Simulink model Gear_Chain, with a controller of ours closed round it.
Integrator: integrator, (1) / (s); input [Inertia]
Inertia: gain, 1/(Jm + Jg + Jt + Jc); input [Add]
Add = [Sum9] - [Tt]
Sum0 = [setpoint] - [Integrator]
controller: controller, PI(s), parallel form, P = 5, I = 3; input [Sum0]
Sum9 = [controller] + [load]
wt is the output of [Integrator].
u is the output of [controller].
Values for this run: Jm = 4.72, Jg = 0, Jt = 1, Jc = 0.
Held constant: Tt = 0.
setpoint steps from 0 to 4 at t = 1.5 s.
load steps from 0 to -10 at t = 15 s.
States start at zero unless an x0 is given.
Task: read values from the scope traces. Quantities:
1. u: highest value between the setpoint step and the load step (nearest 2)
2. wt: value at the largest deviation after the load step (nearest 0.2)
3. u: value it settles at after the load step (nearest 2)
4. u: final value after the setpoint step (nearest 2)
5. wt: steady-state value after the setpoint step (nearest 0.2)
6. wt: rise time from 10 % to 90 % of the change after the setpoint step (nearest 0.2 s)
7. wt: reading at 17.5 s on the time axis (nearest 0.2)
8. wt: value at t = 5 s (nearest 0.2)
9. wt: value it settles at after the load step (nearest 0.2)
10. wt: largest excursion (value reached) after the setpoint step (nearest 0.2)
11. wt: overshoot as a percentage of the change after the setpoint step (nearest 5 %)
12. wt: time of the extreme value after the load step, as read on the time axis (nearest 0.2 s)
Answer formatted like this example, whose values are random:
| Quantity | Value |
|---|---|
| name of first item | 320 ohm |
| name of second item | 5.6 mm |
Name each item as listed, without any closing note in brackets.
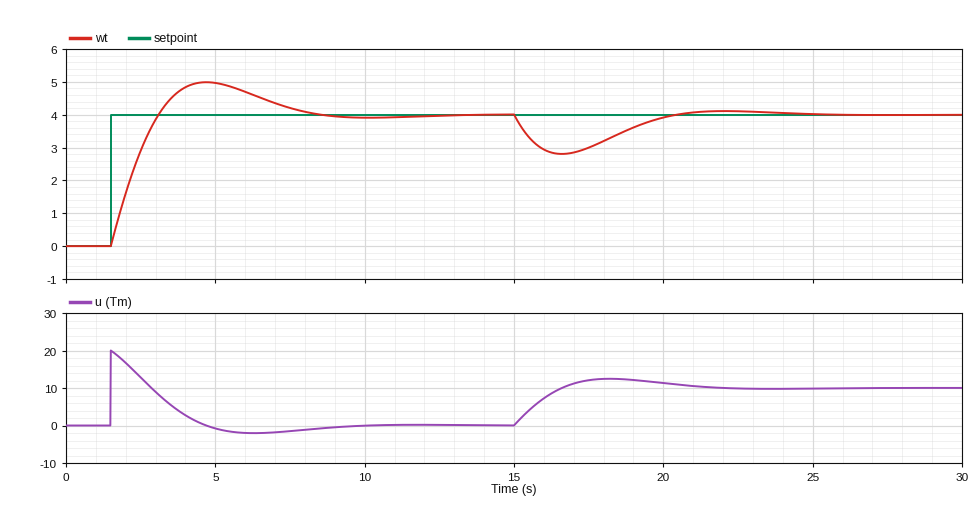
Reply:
| Quantity | Value |
|---|---|
| u: highest value between the setpoint step and the load step | 20 |
| wt: value at the largest deviation after the load step | 2.8 |
| u: value it settles at after the load step | 10 |
| u: final value after the setpoint step | 0 |
| wt: steady-state value after the setpoint step | 4.0 |
| wt: rise time from 10 % to 90 % of the change after the setpoint step | 1.2 s |
| wt: reading at 17.5 s on the time axis | 3.0 |
| wt: value at t = 5 s | 5.0 |
| wt: value it settles at after the load step | 4.0 |
| wt: largest excursion (value reached) after the setpoint step | 5.0 |
| wt: overshoot as a percentage of the change after the setpoint step | 25 % |
| wt: time of the extreme value after the load step, as read on the time axis | 16.6 s |
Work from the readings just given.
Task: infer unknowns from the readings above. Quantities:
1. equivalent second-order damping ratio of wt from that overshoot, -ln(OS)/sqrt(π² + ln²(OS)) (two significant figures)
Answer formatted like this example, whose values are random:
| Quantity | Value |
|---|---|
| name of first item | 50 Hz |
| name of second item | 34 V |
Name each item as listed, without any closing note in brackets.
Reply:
| Quantity | Value |
|---|---|
| equivalent second-order damping ratio of wt from that overshoot, -ln(OS)/sqrt(π² + ln²(OS)) | 0.40 |
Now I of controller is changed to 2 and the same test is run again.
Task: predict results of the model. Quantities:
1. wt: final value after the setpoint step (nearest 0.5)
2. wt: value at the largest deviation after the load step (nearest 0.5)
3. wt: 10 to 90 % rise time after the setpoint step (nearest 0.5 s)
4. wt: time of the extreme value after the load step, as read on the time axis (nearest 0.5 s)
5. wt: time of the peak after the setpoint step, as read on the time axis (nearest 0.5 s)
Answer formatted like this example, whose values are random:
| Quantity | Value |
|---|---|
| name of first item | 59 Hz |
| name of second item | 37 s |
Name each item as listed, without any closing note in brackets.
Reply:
| Quantity | Value |
|---|---|
| wt: final value after the setpoint step | 4.0 |
| wt: value at the largest deviation after the load step | 2.5 |
| wt: 10 to 90 % rise time after the setpoint step | 1.5 s |
| wt: time of the extreme value after the load step, as read on the time axis | 17.0 s |
| wt: time of the peak after the setpoint step, as read on the time axis | 5.0 s |
